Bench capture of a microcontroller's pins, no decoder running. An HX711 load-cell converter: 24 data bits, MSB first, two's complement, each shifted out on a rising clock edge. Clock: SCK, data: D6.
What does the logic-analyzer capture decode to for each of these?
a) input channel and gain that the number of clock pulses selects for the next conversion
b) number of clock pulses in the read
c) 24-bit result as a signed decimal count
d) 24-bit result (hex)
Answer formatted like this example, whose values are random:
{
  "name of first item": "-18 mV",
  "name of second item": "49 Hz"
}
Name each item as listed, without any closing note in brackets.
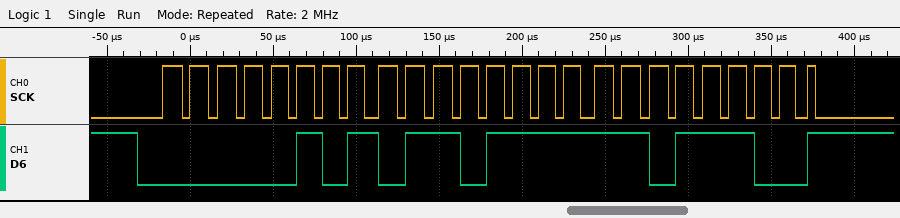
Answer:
{
  "input channel and gain that the number of clock pulses selects for the next conversion": "channel A, gain 128",
  "number of clock pulses in the read": "25",
  "24-bit result as a signed decimal count": "356316",
  "24-bit result": "0x056FDC"
}
